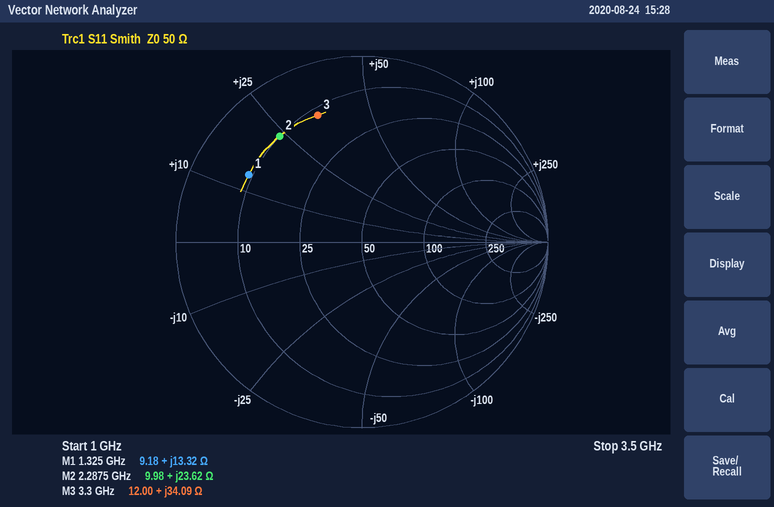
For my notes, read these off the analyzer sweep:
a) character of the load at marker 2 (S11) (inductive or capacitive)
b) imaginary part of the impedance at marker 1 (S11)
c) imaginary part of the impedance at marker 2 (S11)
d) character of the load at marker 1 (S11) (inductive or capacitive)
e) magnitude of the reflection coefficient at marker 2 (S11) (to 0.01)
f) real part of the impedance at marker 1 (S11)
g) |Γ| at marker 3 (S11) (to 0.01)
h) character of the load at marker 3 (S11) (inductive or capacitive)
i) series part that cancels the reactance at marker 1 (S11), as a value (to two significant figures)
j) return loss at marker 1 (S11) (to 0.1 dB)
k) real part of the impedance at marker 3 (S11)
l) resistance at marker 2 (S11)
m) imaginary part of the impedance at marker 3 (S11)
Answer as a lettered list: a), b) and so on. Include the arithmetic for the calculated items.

a) inductive
b) +13.32 Ω
c) +23.62 Ω
d) inductive
e) 0.72
f) 9.18 Ω
g) 0.72
h) inductive
i) C = 1/(2π × 1.325 GHz × 13.32 Ω) ≈ 9.0 pF
j) 3.0 dB
k) 12.00 Ω
l) 9.98 Ω
m) +34.09 Ω
